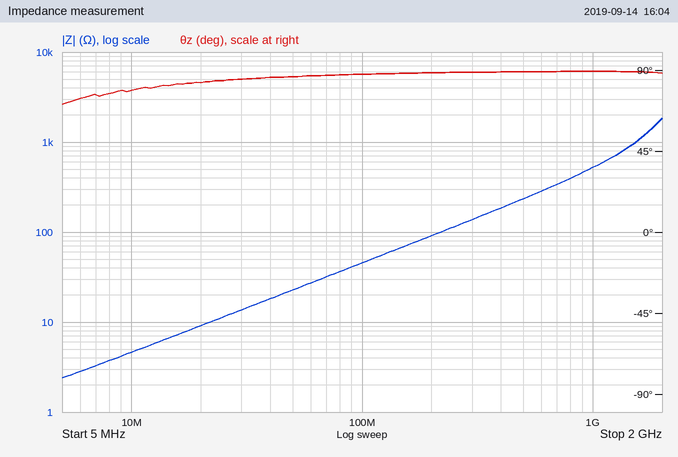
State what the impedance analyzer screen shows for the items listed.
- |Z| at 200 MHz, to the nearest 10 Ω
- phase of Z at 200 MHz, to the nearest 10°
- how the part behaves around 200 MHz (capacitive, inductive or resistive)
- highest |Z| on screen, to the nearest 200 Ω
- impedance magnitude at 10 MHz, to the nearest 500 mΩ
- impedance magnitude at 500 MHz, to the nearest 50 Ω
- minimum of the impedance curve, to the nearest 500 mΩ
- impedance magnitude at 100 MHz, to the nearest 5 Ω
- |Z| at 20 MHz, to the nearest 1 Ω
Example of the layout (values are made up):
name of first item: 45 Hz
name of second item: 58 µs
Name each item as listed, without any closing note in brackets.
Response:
|Z| at 200 MHz, to the nearest 10 Ω: 90 Ω
phase of Z at 200 MHz, to the nearest 10°: 90°
how the part behaves around 200 MHz: inductive
highest |Z| on screen, to the nearest 200 Ω: 1.8 kΩ
impedance magnitude at 10 MHz, to the nearest 500 mΩ: 4.5 Ω
impedance magnitude at 500 MHz, to the nearest 50 Ω: 250 Ω
minimum of the impedance curve, to the nearest 500 mΩ: 2.5 Ω
impedance magnitude at 100 MHz, to the nearest 5 Ω: 45 Ω
|Z| at 20 MHz, to the nearest 1 Ω: 9 Ω
